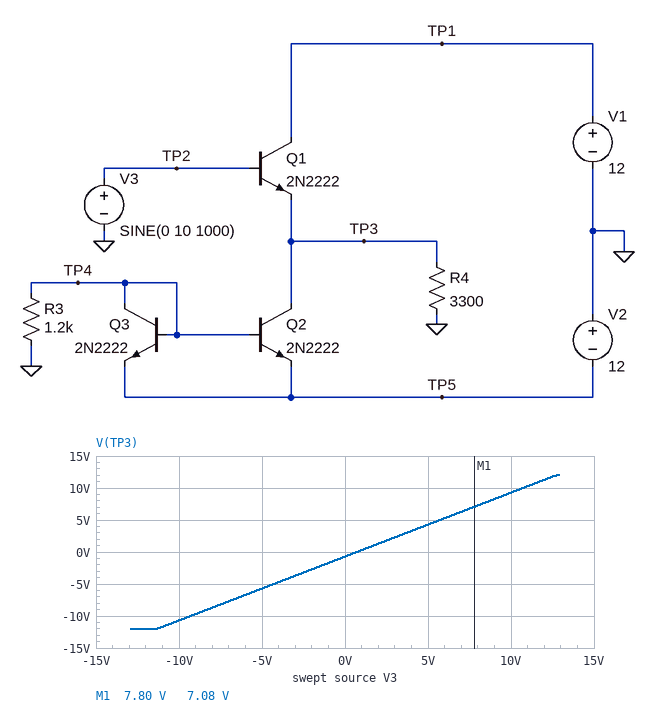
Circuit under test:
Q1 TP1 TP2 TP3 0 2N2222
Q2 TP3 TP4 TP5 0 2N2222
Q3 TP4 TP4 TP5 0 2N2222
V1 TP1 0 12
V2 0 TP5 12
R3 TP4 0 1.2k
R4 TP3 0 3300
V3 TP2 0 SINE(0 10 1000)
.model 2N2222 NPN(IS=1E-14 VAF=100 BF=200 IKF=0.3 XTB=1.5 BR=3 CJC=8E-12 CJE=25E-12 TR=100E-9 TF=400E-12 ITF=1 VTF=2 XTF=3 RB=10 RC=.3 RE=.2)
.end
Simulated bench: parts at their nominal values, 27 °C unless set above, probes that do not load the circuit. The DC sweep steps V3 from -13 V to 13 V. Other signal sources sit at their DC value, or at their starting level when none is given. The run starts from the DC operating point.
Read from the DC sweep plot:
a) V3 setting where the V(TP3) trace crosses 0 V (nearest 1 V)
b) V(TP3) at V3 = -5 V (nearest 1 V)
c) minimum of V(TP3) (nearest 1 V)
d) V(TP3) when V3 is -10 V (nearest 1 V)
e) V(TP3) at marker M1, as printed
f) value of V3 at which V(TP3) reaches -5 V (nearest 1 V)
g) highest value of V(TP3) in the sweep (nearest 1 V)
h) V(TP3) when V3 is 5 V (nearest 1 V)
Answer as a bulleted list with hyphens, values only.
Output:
- 1 V
- -6 V
- -12 V
- -11 V
- 7.08 V
- -4 V
- 12 V
- 4 V
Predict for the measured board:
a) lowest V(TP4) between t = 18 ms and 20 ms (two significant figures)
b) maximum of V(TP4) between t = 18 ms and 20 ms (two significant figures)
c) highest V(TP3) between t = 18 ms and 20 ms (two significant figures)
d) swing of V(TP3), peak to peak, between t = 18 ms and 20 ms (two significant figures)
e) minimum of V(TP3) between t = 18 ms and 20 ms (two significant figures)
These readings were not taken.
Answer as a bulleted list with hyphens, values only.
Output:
- -11 V
- -11 V
- 9.3 V
- 20 V
- -11 V
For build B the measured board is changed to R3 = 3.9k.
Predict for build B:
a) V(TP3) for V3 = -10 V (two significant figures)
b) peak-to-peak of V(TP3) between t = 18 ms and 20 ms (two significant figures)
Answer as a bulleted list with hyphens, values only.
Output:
- -9.6 V
- 19 V
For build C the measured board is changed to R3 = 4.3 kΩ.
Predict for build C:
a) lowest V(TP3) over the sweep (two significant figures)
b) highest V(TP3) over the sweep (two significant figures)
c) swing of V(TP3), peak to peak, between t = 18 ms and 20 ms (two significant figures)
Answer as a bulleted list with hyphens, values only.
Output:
- -8.8 V
- 12 V
- 18 V
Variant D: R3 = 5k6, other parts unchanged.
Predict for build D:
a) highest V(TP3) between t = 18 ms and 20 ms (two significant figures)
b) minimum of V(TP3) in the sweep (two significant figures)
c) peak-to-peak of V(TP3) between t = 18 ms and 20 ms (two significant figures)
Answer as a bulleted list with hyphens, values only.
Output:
- 9.3 V
- -6.9 V
- 16 V
